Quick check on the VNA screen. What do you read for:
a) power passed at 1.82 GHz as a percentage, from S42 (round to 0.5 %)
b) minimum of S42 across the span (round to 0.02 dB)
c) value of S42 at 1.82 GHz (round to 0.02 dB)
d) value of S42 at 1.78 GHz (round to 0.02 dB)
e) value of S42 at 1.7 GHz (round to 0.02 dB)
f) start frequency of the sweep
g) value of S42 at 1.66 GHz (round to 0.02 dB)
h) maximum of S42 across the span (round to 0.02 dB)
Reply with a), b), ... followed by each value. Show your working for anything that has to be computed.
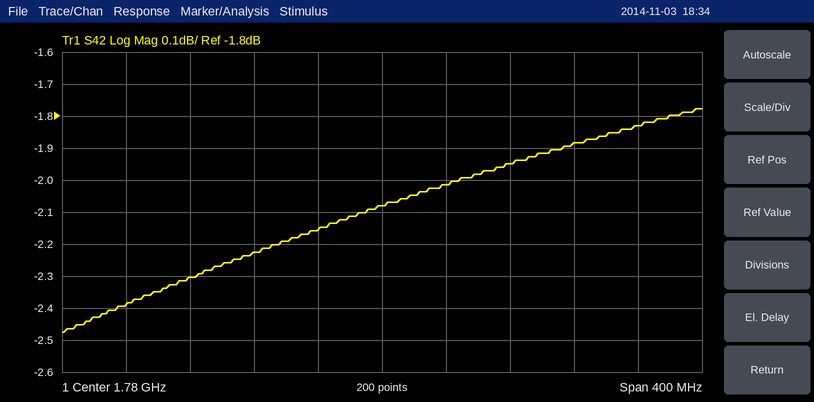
a) 10^(-2.02/10) ≈ 62.8 %, so 63.0 % to the nearest 0.5 %
b) -2.48 dB
c) -2.02 dB
d) -2.08 dB
e) -2.22 dB
f) 1.58 GHz
g) -2.30 dB
h) -1.78 dB
